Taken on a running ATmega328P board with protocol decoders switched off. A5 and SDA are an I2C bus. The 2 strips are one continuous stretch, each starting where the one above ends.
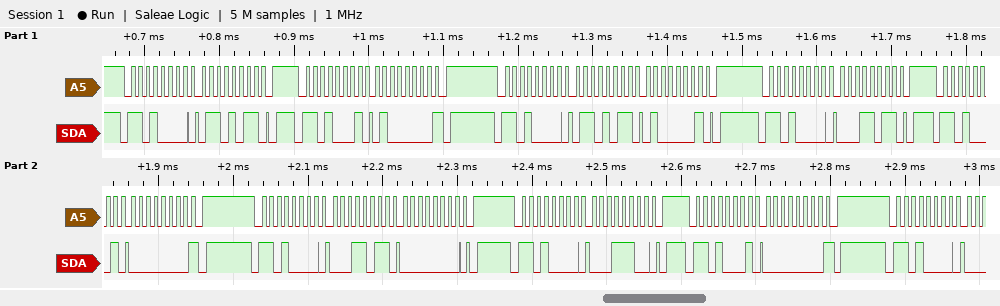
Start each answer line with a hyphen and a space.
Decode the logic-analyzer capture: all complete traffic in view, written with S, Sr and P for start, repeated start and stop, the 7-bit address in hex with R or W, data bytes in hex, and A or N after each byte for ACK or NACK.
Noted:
- S 68W A 6B A P S 68R A 40 N P S 68W A 6B A 41 A P S 68W A 1B A P S 68R A 00 N P S 68W A 1B A 00 A P S 68W A 1C A P S 68R A 00 N P S 68W A
